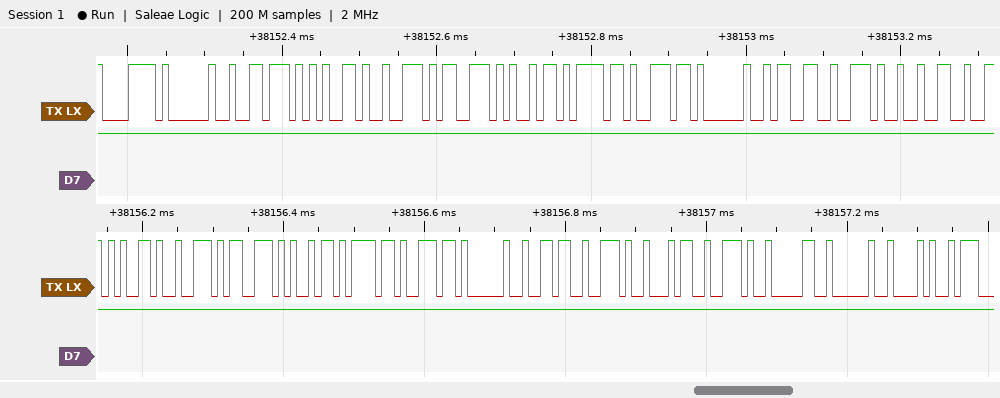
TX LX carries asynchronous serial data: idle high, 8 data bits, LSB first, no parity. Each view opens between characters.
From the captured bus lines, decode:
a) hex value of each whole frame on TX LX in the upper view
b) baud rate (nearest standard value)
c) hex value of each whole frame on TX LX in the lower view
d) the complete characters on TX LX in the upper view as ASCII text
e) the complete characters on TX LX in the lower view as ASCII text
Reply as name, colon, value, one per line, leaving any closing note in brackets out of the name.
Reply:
hex value of each whole frame on TX LX in the upper view: 78, 20, 76, 65, 72, 73, 69, 6F, 6E, 20, 33, 2E, 32
baud rate: 115200 baud
hex value of each whole frame on TX LX in the lower view: 65, 72, 73, 69, 6F, 6E, 20, 36, 2E, 34, 2E, 30, 20, 28
the complete characters on TX LX in the upper view as ASCII text: "x version 3.2"
the complete characters on TX LX in the lower view as ASCII text: "ersion 6.4.0 ("
